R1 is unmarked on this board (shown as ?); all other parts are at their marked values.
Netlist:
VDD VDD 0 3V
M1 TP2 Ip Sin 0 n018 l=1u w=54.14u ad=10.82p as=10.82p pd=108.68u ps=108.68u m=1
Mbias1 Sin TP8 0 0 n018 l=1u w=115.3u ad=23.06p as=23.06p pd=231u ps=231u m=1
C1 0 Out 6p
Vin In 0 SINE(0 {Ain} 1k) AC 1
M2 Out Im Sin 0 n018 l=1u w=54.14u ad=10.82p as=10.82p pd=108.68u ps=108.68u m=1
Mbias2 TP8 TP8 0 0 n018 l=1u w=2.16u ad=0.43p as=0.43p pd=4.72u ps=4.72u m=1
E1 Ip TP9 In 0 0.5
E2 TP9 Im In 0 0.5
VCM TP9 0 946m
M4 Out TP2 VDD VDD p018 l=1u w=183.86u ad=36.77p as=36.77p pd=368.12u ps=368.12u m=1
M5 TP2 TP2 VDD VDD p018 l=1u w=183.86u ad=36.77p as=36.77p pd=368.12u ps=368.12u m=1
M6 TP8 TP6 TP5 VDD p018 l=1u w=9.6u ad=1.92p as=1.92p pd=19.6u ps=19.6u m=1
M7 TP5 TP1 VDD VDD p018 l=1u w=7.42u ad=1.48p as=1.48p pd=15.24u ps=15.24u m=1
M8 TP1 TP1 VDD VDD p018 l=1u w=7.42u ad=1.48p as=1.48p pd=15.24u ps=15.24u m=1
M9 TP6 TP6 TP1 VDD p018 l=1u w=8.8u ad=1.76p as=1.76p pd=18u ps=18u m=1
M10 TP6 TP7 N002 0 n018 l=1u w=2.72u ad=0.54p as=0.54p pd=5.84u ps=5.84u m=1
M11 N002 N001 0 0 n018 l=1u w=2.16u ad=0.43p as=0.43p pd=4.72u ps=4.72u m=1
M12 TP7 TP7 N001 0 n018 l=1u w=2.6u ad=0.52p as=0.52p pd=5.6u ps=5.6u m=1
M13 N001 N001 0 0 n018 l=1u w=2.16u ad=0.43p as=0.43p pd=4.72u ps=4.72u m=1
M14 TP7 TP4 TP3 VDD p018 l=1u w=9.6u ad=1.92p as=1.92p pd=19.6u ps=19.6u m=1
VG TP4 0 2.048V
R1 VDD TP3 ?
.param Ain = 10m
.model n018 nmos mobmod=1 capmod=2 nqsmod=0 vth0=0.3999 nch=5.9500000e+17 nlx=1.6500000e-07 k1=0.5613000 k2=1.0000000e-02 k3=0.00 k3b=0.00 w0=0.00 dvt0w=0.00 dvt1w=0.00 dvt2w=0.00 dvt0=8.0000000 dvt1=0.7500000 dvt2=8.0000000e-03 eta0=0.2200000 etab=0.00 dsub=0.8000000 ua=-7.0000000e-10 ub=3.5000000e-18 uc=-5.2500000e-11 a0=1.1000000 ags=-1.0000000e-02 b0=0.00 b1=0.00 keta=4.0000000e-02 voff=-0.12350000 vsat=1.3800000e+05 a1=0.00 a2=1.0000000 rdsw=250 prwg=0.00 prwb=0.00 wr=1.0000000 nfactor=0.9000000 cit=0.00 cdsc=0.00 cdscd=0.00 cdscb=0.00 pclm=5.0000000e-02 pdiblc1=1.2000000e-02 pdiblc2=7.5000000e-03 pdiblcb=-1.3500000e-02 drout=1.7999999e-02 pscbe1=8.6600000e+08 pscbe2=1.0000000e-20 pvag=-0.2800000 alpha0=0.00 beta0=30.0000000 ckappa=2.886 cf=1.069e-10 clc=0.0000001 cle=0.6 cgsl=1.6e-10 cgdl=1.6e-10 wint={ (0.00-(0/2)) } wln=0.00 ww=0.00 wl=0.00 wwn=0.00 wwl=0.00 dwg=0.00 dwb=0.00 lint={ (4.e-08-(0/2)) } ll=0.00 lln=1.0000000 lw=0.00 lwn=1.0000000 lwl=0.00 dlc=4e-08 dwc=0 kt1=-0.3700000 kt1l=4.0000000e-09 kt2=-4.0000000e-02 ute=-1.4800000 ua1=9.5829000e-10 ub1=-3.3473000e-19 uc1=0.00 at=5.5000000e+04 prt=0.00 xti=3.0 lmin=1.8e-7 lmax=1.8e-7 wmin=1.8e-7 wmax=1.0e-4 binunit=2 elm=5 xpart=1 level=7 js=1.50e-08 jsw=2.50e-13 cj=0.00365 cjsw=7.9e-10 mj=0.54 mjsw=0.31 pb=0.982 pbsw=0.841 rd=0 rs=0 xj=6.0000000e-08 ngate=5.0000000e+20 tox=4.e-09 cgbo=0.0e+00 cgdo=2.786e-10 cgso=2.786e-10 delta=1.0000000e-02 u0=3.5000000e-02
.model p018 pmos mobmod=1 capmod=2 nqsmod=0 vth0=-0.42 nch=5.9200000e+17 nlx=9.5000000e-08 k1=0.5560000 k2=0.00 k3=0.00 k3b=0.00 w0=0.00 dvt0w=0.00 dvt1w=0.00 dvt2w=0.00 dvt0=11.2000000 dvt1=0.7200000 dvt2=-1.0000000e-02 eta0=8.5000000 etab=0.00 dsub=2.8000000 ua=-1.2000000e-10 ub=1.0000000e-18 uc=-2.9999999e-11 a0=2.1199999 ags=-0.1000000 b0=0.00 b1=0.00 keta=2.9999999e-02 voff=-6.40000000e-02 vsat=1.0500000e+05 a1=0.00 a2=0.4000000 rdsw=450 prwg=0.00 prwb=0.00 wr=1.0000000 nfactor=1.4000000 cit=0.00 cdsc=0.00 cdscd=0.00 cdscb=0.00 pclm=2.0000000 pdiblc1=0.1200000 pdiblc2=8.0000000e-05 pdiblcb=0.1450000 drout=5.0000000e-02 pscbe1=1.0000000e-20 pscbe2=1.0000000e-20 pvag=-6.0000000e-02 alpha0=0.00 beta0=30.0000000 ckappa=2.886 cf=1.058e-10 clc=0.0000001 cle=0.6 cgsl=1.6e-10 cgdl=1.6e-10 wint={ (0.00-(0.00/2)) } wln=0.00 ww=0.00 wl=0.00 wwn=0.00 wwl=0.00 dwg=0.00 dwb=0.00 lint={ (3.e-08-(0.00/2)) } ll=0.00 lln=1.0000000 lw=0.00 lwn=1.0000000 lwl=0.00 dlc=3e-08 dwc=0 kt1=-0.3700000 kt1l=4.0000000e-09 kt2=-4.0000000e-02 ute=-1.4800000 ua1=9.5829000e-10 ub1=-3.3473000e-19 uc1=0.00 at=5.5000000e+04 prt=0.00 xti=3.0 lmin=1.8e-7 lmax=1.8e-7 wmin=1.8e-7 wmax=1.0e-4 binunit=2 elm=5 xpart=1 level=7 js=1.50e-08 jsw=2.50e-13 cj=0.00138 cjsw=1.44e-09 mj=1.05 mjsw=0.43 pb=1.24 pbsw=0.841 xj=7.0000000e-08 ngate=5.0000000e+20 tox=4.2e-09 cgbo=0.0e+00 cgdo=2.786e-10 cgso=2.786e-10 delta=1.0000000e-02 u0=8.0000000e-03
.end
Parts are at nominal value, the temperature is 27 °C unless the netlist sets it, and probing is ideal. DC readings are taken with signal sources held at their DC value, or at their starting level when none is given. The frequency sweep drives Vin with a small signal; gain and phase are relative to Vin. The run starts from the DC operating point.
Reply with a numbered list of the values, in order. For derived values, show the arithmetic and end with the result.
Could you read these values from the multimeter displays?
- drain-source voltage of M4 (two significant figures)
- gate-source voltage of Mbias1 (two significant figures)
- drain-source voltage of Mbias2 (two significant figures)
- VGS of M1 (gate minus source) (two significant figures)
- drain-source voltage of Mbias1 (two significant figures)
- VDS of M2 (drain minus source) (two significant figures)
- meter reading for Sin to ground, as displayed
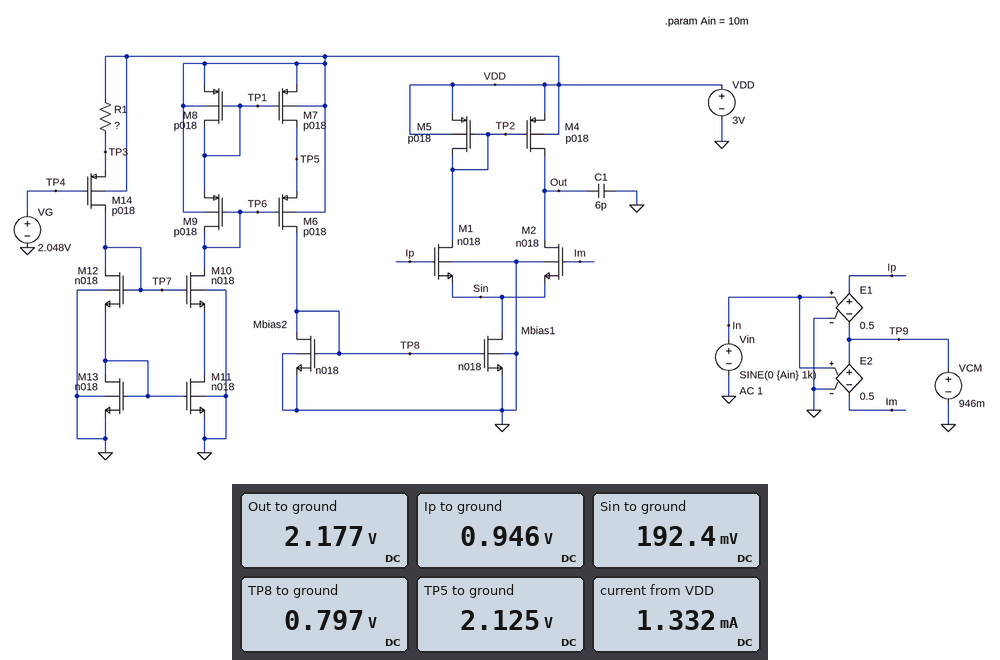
1. 2.177 V - 3 V = -820 mV
2. 797 mV = 800 mV
3. 797 mV = 800 mV
4. 946 mV - 192.4 mV = 750 mV
5. 192.4 mV = 190 mV
6. 2.177 V - 192.4 mV = 2.0 V
7. 192.4 mV
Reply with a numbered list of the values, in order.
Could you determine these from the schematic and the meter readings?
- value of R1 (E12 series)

1. 5.6 kΩ
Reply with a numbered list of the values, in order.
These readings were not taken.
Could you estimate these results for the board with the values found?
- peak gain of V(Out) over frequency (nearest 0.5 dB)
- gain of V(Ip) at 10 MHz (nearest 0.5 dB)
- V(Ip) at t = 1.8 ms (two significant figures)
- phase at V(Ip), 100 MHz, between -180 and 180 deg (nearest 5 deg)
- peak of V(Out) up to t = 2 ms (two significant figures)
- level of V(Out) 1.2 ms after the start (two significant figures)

1. 30.5 dB
2. -6.0 dB
3. 940 mV
4. 0 deg
5. 2.4 V
6. 2.4 V
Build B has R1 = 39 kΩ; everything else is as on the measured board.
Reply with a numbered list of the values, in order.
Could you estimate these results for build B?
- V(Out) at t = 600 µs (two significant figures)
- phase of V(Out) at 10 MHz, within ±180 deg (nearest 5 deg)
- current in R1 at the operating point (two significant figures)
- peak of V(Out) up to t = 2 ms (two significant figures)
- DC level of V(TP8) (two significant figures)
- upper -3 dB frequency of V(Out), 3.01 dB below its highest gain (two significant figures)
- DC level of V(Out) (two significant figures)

1. 2.0 V
2. -85 deg
3. 7.8 µA
4. 2.6 V
5. 610 mV
6. 1.4 MHz
7. 2.3 V
